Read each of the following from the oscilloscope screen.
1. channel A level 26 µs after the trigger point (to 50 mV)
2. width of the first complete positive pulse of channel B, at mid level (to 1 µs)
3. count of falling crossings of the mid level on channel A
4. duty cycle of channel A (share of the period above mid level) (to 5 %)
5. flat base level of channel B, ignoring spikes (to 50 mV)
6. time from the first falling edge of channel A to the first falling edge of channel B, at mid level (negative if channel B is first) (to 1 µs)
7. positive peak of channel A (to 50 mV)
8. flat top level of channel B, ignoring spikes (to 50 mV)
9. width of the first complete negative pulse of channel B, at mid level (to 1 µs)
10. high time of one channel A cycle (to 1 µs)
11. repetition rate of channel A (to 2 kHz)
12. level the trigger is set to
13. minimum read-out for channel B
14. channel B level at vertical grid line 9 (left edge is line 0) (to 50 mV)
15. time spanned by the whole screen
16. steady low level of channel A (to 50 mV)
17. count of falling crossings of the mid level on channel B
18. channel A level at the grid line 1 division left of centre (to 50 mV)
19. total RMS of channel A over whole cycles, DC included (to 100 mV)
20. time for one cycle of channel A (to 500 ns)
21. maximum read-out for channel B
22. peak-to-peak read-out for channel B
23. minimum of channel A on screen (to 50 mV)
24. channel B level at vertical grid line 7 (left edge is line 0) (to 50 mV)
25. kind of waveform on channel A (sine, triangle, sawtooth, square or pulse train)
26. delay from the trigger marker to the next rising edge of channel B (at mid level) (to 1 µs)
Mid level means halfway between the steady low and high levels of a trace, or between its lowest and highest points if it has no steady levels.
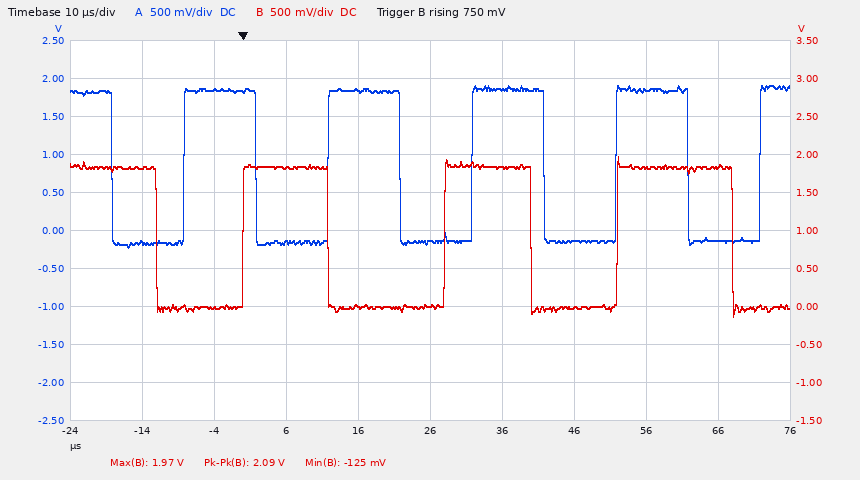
-150 mV
12 µs
5
50 %
0 mV
+6 µs
1.90 V
1.85 V
12 µs
10 µs
50 kHz
750 mV
-125 mV
1.85 V
100 µs
-150 mV
4
1.85 V
1.3 V
20.0 µs
1.97 V
2.09 V
-200 mV
0 mV
square
28 µs
